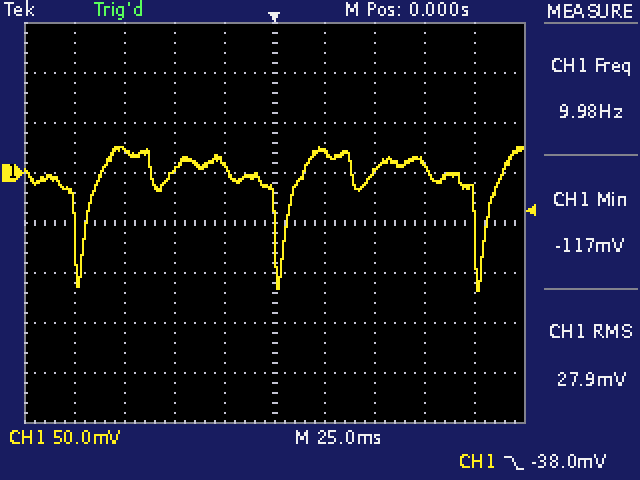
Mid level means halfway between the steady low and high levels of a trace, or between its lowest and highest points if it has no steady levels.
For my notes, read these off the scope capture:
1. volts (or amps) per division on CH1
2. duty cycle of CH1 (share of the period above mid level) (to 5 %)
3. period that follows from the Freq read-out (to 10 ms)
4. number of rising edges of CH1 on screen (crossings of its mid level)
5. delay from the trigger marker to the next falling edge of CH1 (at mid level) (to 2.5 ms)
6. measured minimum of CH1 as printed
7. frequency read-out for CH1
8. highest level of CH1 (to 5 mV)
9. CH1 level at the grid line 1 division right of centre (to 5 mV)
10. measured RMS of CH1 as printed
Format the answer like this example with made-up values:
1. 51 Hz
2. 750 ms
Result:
1. 50 mV
2. 95 %
3. 100 ms
4. 3
5. 100.0 ms
6. -117 mV
7. 9.98 Hz
8. 25 mV
9. 20 mV
10. 27.9 mV
